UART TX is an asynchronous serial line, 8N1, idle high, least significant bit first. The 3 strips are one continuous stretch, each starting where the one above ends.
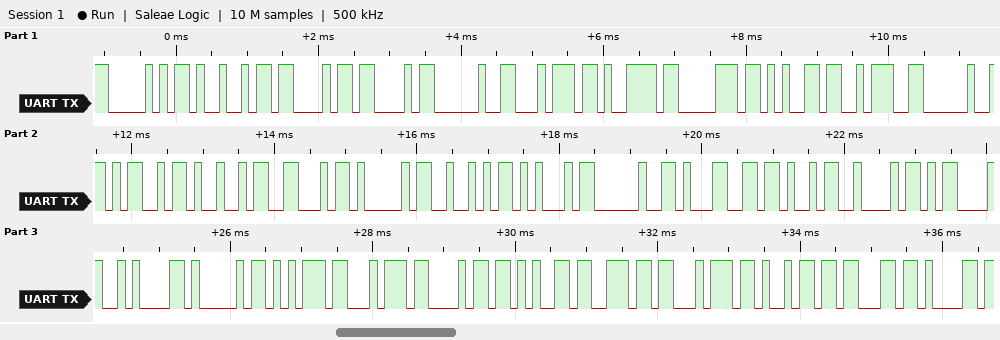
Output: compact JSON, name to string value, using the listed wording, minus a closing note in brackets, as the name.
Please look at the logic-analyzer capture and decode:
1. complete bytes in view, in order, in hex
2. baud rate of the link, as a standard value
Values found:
{"complete bytes in view, in order, in hex": "50 49 43 43 20 74 79 70 65 3A 20 4D 49 46 41 52 45 20 31 4B 42 0D 0A 41 75 74 68 65 6E 74 69 63 61", "baud rate of the link, as a standard value": "9600 baud"}
